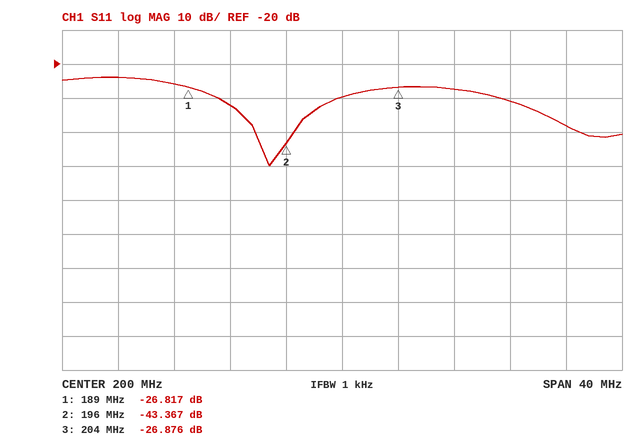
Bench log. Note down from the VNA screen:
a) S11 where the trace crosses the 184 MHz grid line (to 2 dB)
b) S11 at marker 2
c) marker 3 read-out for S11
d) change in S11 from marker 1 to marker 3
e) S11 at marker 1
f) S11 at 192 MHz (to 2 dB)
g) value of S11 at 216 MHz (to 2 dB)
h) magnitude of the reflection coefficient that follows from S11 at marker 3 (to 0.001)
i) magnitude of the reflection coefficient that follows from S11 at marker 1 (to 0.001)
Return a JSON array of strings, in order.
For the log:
["-24 dB", "-43.367 dB", "-26.876 dB", "-0.059 dB", "-26.817 dB", "-32 dB", "-38 dB", "0.045", "0.046"]
